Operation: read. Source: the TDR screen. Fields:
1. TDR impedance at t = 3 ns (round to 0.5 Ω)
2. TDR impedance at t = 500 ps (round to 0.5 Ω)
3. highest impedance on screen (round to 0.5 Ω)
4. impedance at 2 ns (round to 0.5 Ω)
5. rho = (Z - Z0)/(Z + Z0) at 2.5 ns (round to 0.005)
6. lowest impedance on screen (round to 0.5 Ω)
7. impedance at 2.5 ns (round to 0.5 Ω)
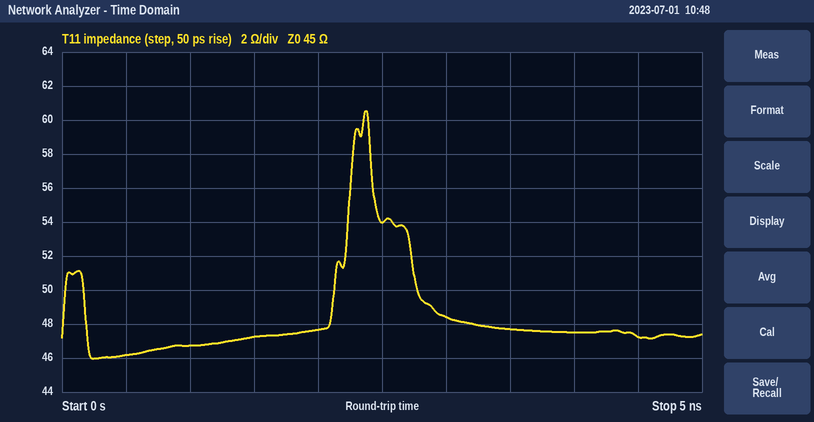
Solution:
48.5 Ω
46.0 Ω
60.5 Ω
47.5 Ω
+0.090
46.0 Ω
54.0 Ω
